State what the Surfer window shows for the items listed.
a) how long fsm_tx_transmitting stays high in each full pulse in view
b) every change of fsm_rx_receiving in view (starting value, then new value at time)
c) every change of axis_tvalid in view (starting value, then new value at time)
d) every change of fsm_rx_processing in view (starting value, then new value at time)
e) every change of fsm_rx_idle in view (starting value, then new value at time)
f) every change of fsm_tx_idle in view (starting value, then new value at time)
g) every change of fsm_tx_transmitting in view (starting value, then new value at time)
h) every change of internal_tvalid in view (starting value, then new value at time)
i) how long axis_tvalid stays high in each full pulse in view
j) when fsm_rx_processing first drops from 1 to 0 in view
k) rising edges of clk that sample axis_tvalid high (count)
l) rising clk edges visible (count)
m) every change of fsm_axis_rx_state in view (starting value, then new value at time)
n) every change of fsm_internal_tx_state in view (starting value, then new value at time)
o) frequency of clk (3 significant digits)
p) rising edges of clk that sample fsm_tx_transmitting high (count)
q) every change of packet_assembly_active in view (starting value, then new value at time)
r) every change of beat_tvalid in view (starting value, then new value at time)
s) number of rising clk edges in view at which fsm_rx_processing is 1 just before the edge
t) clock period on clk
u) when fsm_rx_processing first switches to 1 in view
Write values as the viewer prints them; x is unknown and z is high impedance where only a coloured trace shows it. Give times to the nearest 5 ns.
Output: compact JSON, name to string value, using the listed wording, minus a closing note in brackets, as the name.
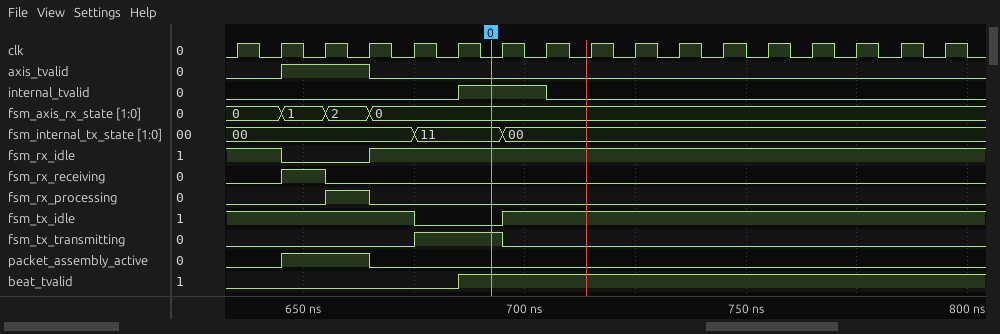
{"how long fsm_tx_transmitting stays high in each full pulse in view": "20 ns", "every change of fsm_rx_receiving in view": "0, 1 at 645 ns, 0 at 655 ns", "every change of axis_tvalid in view": "0, 1 at 645 ns, 0 at 665 ns", "every change of fsm_rx_processing in view": "0, 1 at 655 ns, 0 at 665 ns", "every change of fsm_rx_idle in view": "1, 0 at 645 ns, 1 at 665 ns", "every change of fsm_tx_idle in view": "1, 0 at 675 ns, 1 at 695 ns", "every change of fsm_tx_transmitting in view": "0, 1 at 675 ns, 0 at 695 ns", "every change of internal_tvalid in view": "0, 1 at 685 ns, 0 at 705 ns", "how long axis_tvalid stays high in each full pulse in view": "20 ns", "when fsm_rx_processing first drops from 1 to 0 in view": "665 ns", "rising edges of clk that sample axis_tvalid high": "2", "rising clk edges visible": "17", "every change of fsm_axis_rx_state in view": "0, 1 at 645 ns, 2 at 655 ns, 0 at 665 ns", "every change of fsm_internal_tx_state in view": "00, 11 at 675 ns, 00 at 695 ns", "frequency of clk": "100 MHz", "rising edges of clk that sample fsm_tx_transmitting high": "2", "every change of packet_assembly_active in view": "0, 1 at 645 ns, 0 at 665 ns", "every change of beat_tvalid in view": "0, 1 at 685 ns", "number of rising clk edges in view at which fsm_rx_processing is 1 just before the edge": "1", "clock period on clk": "10 ns", "when fsm_rx_processing first switches to 1 in view": "655 ns"}
